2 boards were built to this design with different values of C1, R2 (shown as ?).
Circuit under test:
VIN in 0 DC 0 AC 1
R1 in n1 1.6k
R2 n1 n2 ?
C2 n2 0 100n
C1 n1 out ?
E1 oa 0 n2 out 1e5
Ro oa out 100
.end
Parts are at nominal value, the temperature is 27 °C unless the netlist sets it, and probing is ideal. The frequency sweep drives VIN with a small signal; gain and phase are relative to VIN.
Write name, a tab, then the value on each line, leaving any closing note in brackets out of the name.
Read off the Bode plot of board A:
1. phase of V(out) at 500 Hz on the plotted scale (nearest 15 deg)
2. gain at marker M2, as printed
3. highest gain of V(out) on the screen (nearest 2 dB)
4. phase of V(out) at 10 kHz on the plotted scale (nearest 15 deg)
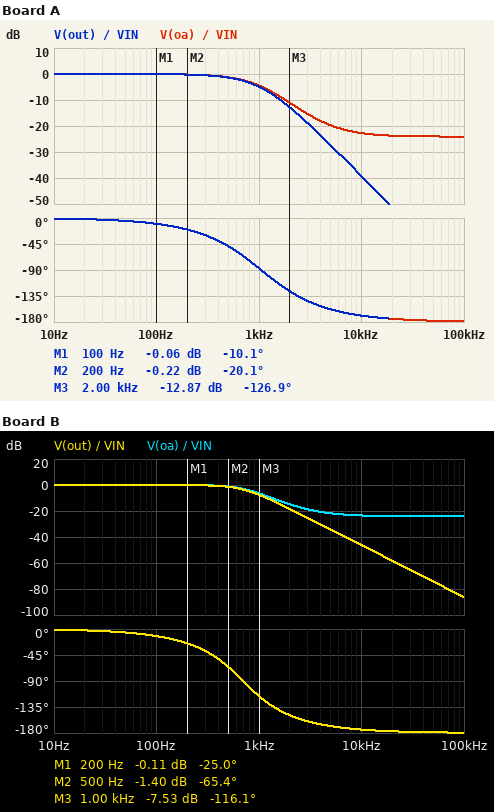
phase of V(out) at 500 Hz on the plotted scale	-45 deg
gain at marker M2, as printed	-0.22 dB
highest gain of V(out) on the screen	0 dB
phase of V(out) at 10 kHz on the plotted scale	-165 deg
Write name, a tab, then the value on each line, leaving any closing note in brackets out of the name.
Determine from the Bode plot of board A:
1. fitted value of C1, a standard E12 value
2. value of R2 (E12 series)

fitted value of C1, a standard E12 value	120 nF
value of R2	1.2 kΩ
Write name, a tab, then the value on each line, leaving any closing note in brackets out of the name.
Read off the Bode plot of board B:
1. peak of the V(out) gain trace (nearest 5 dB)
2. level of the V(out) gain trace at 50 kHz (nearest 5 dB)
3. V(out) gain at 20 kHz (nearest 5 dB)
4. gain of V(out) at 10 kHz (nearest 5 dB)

peak of the V(out) gain trace	0 dB
level of the V(out) gain trace at 50 kHz	-75 dB
V(out) gain at 20 kHz	-60 dB
gain of V(out) at 10 kHz	-45 dB
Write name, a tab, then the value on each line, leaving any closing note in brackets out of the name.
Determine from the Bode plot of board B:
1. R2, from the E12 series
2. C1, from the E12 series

R2, from the E12 series	1.8 kΩ
C1, from the E12 series	180 nF
